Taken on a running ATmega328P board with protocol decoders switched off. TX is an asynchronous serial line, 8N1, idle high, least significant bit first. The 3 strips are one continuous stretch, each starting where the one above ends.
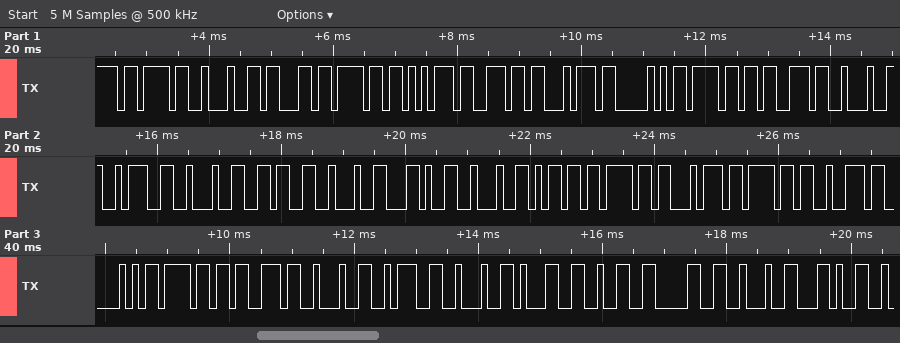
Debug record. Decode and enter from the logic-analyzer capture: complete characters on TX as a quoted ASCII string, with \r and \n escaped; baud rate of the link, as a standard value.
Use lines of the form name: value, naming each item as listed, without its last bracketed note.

complete characters on TX as a quoted ASCII string, with \r and \n escaped: "{\"countPos\":\"6\",\"motorPos\":\"120\","
baud rate of the link, as a standard value: 9600 baud
